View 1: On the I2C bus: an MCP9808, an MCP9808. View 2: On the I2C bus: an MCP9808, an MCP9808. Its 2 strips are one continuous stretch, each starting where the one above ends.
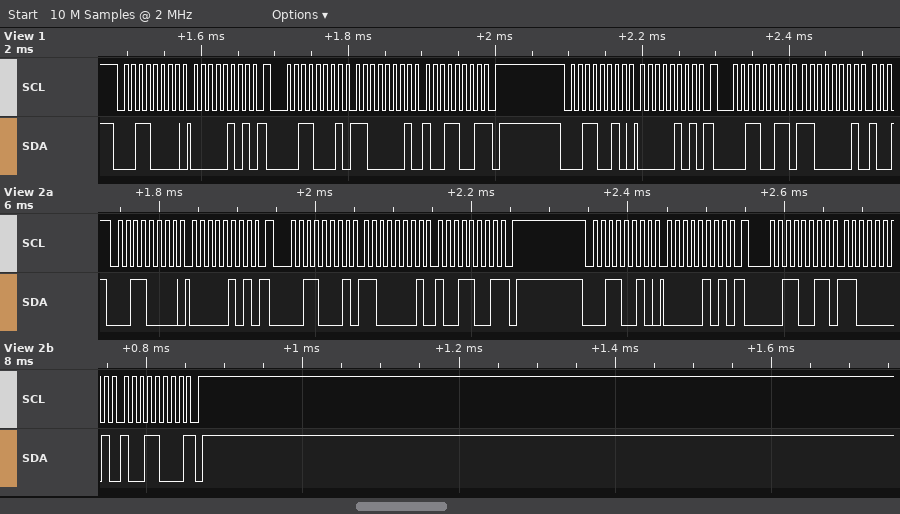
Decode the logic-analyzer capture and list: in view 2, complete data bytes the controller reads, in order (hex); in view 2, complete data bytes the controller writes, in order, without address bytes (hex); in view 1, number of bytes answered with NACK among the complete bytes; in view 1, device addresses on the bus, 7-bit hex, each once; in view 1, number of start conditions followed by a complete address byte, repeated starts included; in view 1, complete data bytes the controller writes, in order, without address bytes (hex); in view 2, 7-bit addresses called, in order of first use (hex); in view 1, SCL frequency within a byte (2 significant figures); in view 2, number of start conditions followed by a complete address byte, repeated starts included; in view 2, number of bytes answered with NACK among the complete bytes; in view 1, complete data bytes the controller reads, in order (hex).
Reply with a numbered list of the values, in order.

1. C1 99 C1 98
2. 05 05
3. 1
4. 0x18 0x19
5. 4
6. 05 05
7. 0x18 0x19
8. 100 kHz
9. 4
10. 2
11. C1 99 C1
